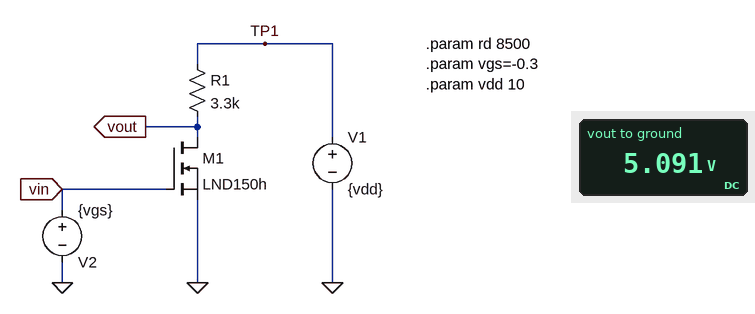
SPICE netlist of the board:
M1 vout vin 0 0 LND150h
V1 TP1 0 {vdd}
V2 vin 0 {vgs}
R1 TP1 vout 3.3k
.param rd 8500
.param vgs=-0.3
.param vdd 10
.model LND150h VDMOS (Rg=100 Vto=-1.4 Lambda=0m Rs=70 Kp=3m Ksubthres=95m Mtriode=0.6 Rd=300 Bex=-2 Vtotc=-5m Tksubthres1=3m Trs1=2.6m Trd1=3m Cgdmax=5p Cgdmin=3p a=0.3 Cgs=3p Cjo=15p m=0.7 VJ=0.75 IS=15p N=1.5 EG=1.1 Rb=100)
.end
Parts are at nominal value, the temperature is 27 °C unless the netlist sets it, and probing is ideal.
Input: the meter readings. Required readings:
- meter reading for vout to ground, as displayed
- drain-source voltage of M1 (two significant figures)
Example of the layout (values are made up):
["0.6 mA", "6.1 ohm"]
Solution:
["5.091 V", "5.1 V"]
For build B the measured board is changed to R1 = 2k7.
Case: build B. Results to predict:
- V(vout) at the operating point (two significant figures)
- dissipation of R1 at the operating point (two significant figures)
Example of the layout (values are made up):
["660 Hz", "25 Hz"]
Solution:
["6.0 V", "6.0 mW"]
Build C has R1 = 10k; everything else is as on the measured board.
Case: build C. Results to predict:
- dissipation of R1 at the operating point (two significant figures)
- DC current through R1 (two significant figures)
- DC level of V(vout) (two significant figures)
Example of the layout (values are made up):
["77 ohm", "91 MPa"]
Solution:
["8.2 mW", "910 µA", "920 mV"]
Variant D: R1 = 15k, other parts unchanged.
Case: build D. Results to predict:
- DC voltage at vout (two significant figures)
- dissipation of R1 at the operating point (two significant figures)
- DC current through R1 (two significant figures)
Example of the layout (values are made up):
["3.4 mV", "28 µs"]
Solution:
["600 mV", "5.9 mW", "630 µA"]
